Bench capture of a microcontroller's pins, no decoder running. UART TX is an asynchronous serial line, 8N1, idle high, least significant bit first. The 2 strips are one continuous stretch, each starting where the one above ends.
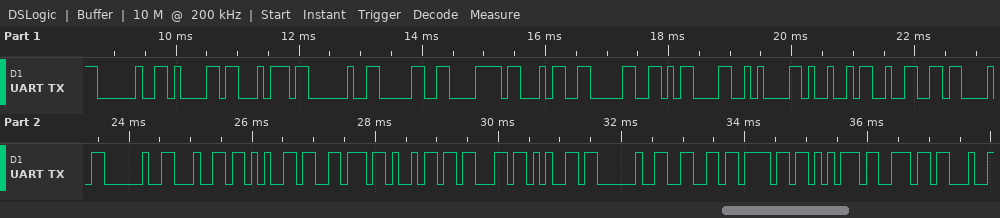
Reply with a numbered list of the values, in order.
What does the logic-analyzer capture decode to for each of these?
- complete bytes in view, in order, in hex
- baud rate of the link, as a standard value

1. 20 61 74 20 30 78 34 30 0D 0A 49 32 43 20 64 65 76 69 63 65 20 66 6F 75 6E
2. 9600 baud
